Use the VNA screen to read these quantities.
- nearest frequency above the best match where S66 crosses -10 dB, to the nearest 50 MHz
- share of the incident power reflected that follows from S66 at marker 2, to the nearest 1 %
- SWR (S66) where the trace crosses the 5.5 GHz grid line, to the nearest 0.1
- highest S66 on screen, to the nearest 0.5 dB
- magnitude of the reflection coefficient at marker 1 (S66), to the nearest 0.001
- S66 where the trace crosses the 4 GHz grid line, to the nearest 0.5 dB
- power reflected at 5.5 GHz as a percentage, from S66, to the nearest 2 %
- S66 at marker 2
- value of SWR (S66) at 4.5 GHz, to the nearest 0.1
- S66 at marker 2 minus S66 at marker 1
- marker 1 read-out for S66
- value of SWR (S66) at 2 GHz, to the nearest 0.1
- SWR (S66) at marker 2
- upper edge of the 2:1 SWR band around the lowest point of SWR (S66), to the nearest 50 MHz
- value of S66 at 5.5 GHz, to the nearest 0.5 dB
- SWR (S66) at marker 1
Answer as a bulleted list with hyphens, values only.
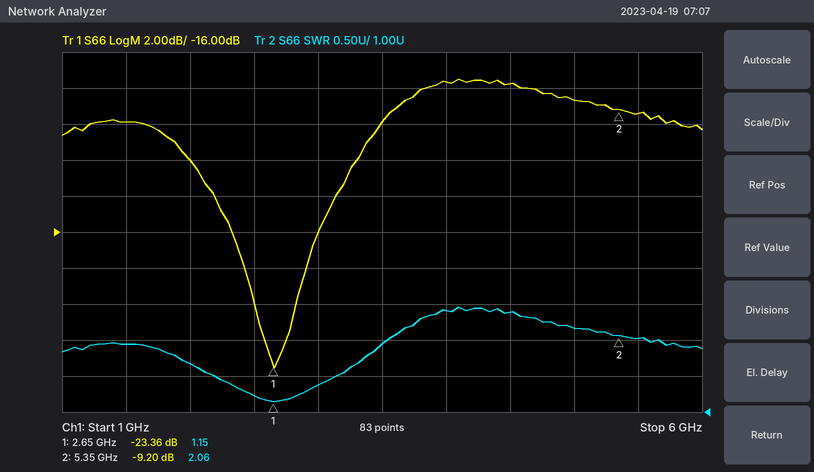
- 3.50 GHz
- 12 %
- 2.0
- -7.5 dB
- 0.068
- -7.5 dB
- 12 %
- -9.20 dB
- 2.4
- 14.16 dB
- -23.36 dB
- 1.7
- 2.06
- 3.55 GHz
- -9.5 dB
- 1.15
